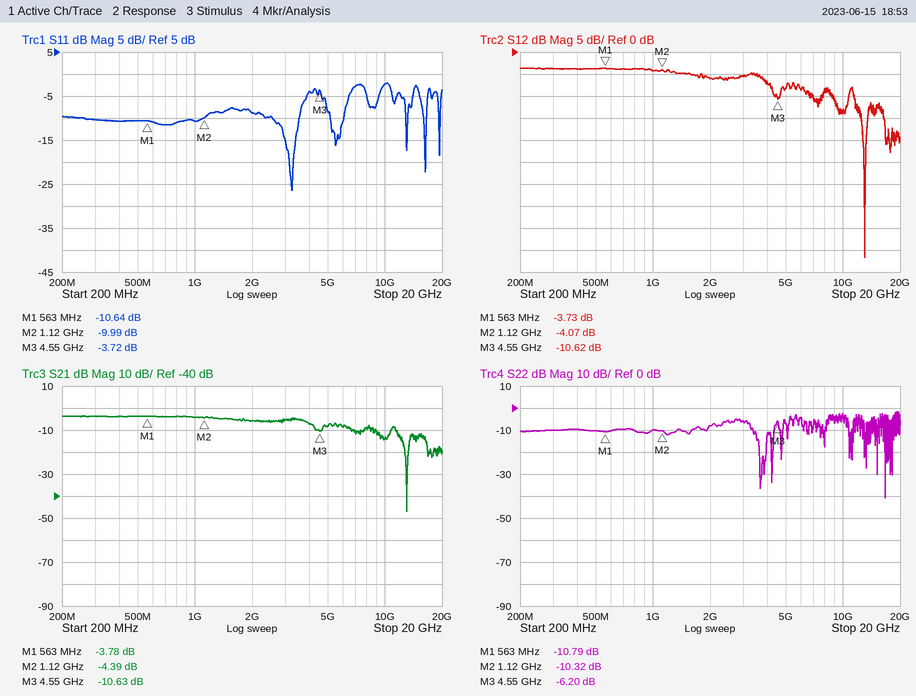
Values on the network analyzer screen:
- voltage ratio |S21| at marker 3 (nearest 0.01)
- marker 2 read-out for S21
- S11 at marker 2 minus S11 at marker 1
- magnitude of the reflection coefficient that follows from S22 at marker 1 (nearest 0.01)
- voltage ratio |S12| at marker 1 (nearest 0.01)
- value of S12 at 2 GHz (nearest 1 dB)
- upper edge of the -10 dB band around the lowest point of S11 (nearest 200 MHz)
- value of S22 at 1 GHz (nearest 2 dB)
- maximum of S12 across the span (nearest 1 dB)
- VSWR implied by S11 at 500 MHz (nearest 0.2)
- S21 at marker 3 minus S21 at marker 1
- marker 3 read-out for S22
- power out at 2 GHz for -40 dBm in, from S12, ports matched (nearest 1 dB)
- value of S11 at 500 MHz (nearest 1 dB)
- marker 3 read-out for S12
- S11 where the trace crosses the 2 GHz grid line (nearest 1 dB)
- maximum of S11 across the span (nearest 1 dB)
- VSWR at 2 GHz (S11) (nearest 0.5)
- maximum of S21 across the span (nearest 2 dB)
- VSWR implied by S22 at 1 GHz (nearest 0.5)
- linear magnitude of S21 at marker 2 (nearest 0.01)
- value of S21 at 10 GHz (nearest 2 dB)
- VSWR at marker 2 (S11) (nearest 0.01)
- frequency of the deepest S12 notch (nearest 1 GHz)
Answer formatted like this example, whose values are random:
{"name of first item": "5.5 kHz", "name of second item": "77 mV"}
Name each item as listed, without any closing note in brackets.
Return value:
{"voltage ratio |S21| at marker 3": "0.29", "marker 2 read-out for S21": "-4.39 dB", "S11 at marker 2 minus S11 at marker 1": "0.65 dB", "magnitude of the reflection coefficient that follows from S22 at marker 1": "0.29", "voltage ratio |S12| at marker 1": "0.65", "value of S12 at 2 GHz": "-6 dB", "upper edge of the -10 dB band around the lowest point of S11": "3.6 GHz", "value of S22 at 1 GHz": "-10 dB", "maximum of S12 across the span": "-4 dB", "VSWR implied by S11 at 500 MHz": "1.8", "S21 at marker 3 minus S21 at marker 1": "-6.85 dB", "marker 3 read-out for S22": "-6.20 dB", "power out at 2 GHz for -40 dBm in, from S12, ports matched": "-46 dBm", "value of S11 at 500 MHz": "-11 dB", "marker 3 read-out for S12": "-10.62 dB", "S11 where the trace crosses the 2 GHz grid line": "-9 dB", "maximum of S11 across the span": "-2 dB", "VSWR at 2 GHz (S11)": "2.0", "maximum of S21 across the span": "-4 dB", "VSWR implied by S22 at 1 GHz": "2.0", "linear magnitude of S21 at marker 2": "0.60", "value of S21 at 10 GHz": "-14 dB", "VSWR at marker 2 (S11)": "1.93", "frequency of the deepest S12 notch": "13 GHz"}
